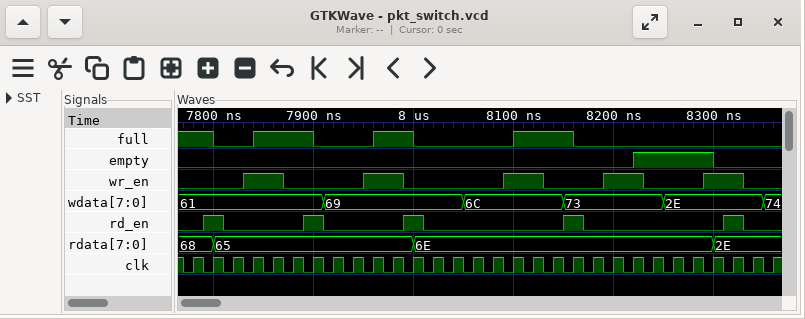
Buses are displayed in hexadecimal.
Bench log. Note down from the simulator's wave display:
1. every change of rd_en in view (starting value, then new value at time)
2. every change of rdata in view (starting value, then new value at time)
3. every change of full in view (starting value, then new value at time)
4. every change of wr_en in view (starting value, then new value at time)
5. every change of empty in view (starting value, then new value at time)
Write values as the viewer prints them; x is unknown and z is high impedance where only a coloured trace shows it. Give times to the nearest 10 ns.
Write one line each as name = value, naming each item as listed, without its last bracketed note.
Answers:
every change of rd_en in view = 0, 1 at 7790 ns, 0 at 7810 ns, 1 at 7890 ns, 0 at 7910 ns, 1 at 7990 ns, 0 at 8010 ns, 1 at 8150 ns, 0 at 8170 ns, 1 at 8310 ns, 0 at 8330 ns
every change of rdata in view = 68, 65 at 7800 ns, 6E at 8000 ns, 2E at 8300 ns
every change of full in view = 1, 0 at 7800 ns, 1 at 7840 ns, 0 at 7900 ns, 1 at 7960 ns, 0 at 8000 ns, 1 at 8100 ns, 0 at 8160 ns
every change of wr_en in view = 0, 1 at 7830 ns, 0 at 7870 ns, 1 at 7950 ns, 0 at 7990 ns, 1 at 8090 ns, 0 at 8130 ns, 1 at 8190 ns, 0 at 8230 ns, 1 at 8290 ns, 0 at 8330 ns
every change of empty in view = 0, 1 at 8220 ns, 0 at 8300 ns
